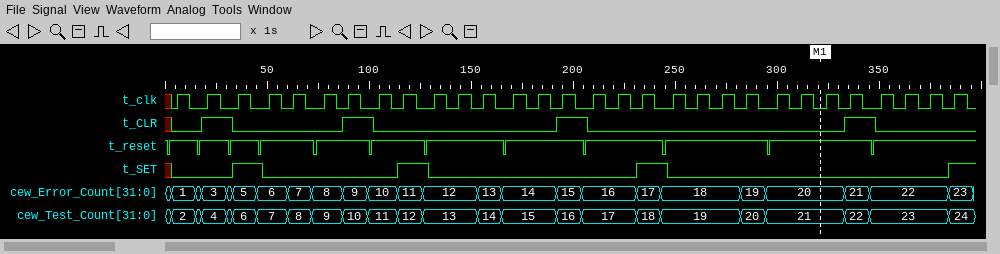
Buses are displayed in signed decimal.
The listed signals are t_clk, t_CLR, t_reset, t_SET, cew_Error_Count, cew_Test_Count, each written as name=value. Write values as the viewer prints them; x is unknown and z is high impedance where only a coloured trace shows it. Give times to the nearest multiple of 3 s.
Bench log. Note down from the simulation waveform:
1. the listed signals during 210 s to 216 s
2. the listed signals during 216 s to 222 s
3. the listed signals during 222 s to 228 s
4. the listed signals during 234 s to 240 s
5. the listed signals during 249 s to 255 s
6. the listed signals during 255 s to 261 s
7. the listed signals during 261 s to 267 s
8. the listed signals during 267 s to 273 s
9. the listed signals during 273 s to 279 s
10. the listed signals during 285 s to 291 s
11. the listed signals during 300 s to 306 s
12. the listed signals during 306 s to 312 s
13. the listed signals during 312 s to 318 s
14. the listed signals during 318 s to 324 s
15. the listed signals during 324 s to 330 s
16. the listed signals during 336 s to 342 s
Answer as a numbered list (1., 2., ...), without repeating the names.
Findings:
1. t_clk=1, t_CLR=0, t_reset=1, t_SET=0, cew_Error_Count=16, cew_Test_Count=17
2. t_clk=0, t_CLR=0, t_reset=1, t_SET=0, cew_Error_Count=16, cew_Test_Count=17
3. t_clk=1, t_CLR=0, t_reset=1, t_SET=0, cew_Error_Count=16, cew_Test_Count=17
4. t_clk=1, t_CLR=0, t_reset=1, t_SET=1, cew_Error_Count=17, cew_Test_Count=18
5. t_clk=1, t_CLR=0, t_reset=1, t_SET=0, cew_Error_Count=18, cew_Test_Count=19
6. t_clk=0, t_CLR=0, t_reset=1, t_SET=0, cew_Error_Count=18, cew_Test_Count=19
7. t_clk=1, t_CLR=0, t_reset=1, t_SET=0, cew_Error_Count=18, cew_Test_Count=19
8. t_clk=0, t_CLR=0, t_reset=1, t_SET=0, cew_Error_Count=18, cew_Test_Count=19
9. t_clk=1, t_CLR=0, t_reset=1, t_SET=0, cew_Error_Count=18, cew_Test_Count=19
10. t_clk=1, t_CLR=0, t_reset=1, t_SET=0, cew_Error_Count=19, cew_Test_Count=20
11. t_clk=1, t_CLR=0, t_reset=1, t_SET=0, cew_Error_Count=20, cew_Test_Count=21
12. t_clk=0, t_CLR=0, t_reset=1, t_SET=0, cew_Error_Count=20, cew_Test_Count=21
13. t_clk=1, t_CLR=0, t_reset=1, t_SET=0, cew_Error_Count=20, cew_Test_Count=21
14. t_clk=0, t_CLR=0, t_reset=1, t_SET=0, cew_Error_Count=20, cew_Test_Count=21
15. t_clk=1, t_CLR=0, t_reset=1, t_SET=0, cew_Error_Count=20, cew_Test_Count=21
16. t_clk=1, t_CLR=1, t_reset=1, t_SET=0, cew_Error_Count=21, cew_Test_Count=22
